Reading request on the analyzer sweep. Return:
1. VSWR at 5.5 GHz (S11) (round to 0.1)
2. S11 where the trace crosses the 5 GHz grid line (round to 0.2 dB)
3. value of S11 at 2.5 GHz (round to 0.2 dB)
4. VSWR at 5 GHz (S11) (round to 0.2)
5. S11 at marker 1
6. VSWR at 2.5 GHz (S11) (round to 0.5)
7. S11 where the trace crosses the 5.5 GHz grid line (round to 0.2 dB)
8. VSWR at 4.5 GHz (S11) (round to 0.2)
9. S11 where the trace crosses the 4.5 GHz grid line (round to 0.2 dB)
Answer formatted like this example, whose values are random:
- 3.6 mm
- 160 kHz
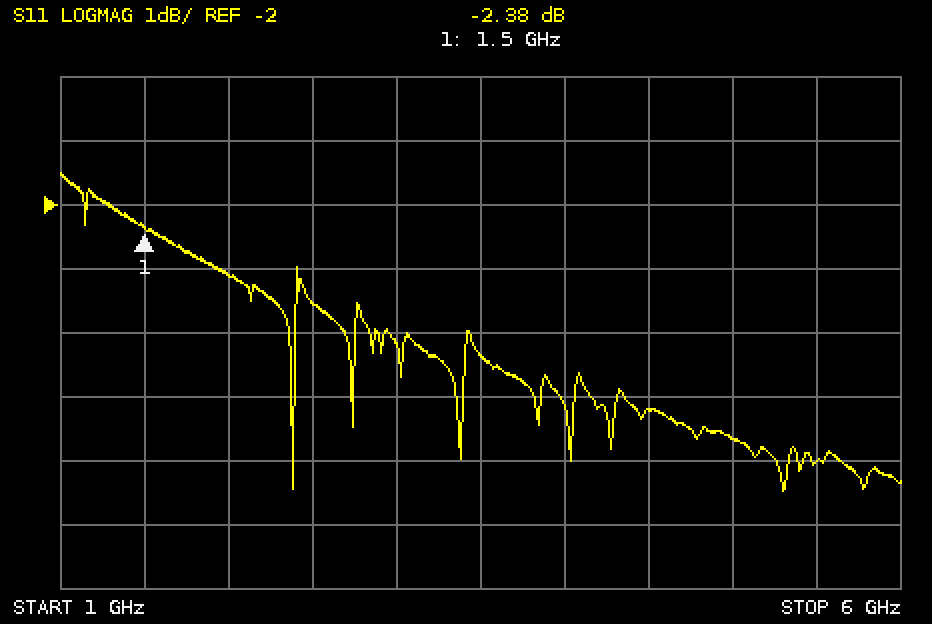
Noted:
- 3.0
- -5.6 dB
- -3.6 dB
- 3.2
- -2.38 dB
- 5.0
- -6.0 dB
- 3.4
- -5.2 dB
